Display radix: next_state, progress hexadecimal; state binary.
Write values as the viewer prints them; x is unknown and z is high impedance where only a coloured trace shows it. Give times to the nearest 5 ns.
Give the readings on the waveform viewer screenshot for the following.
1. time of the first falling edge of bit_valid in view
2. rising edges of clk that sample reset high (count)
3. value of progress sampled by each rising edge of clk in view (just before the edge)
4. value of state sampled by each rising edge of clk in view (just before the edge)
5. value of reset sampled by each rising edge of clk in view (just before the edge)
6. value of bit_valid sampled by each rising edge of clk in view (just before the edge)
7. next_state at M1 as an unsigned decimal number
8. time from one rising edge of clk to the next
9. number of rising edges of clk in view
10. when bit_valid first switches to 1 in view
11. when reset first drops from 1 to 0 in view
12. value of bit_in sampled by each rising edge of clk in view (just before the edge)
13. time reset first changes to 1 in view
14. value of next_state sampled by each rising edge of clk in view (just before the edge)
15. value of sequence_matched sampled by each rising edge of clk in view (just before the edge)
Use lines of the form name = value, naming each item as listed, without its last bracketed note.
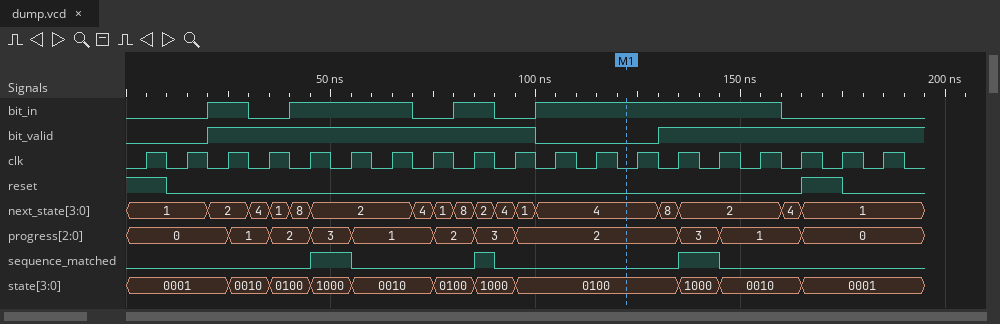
time of the first falling edge of bit_valid in view = 100 ns
rising edges of clk that sample reset high = 2
value of progress sampled by each rising edge of clk in view = 0, 0, 0, 1, 2, 3, 1, 1, 2, 3, 2, 2, 2, 2, 3, 1, 1, 0, 0
value of state sampled by each rising edge of clk in view = 0001, 0001, 0001, 0010, 0100, 1000, 0010, 0010, 0100, 1000, 0100, 0100, 0100, 0100, 1000, 0010, 0010, 0001, 0001
value of reset sampled by each rising edge of clk in view = 1 0 0 0 0 0 0 0 0 0 0 0 0 0 0 0 0 1 0
value of bit_valid sampled by each rising edge of clk in view = 0 0 1 1 1 1 1 1 1 1 0 0 0 1 1 1 1 1 1
next_state at M1 as an unsigned decimal number = 4
time from one rising edge of clk to the next = 10 ns
number of rising edges of clk in view = 19
when bit_valid first switches to 1 in view = 20 ns
when reset first drops from 1 to 0 in view = 10 ns
value of bit_in sampled by each rising edge of clk in view = 0 0 1 0 1 1 1 0 1 0 1 1 1 1 1 1 0 0 0
time reset first changes to 1 in view = 165 ns
value of next_state sampled by each rising edge of clk in view = 1, 1, 2, 4, 8, 2, 2, 4, 8, 4, 4, 4, 4, 8, 2, 2, 4, 1, 1
value of sequence_matched sampled by each rising edge of clk in view = 0 0 0 0 0 1 0 0 0 0 0 0 0 0 1 0 0 0 0
